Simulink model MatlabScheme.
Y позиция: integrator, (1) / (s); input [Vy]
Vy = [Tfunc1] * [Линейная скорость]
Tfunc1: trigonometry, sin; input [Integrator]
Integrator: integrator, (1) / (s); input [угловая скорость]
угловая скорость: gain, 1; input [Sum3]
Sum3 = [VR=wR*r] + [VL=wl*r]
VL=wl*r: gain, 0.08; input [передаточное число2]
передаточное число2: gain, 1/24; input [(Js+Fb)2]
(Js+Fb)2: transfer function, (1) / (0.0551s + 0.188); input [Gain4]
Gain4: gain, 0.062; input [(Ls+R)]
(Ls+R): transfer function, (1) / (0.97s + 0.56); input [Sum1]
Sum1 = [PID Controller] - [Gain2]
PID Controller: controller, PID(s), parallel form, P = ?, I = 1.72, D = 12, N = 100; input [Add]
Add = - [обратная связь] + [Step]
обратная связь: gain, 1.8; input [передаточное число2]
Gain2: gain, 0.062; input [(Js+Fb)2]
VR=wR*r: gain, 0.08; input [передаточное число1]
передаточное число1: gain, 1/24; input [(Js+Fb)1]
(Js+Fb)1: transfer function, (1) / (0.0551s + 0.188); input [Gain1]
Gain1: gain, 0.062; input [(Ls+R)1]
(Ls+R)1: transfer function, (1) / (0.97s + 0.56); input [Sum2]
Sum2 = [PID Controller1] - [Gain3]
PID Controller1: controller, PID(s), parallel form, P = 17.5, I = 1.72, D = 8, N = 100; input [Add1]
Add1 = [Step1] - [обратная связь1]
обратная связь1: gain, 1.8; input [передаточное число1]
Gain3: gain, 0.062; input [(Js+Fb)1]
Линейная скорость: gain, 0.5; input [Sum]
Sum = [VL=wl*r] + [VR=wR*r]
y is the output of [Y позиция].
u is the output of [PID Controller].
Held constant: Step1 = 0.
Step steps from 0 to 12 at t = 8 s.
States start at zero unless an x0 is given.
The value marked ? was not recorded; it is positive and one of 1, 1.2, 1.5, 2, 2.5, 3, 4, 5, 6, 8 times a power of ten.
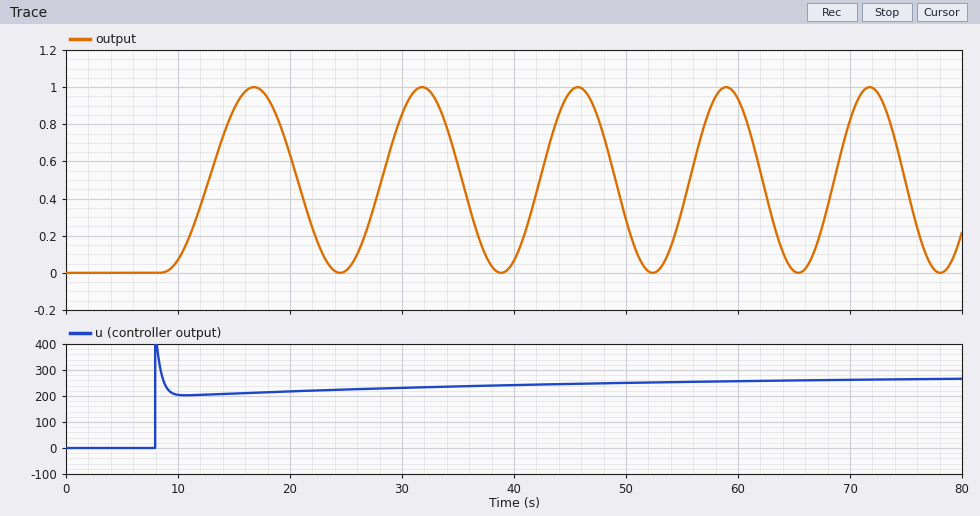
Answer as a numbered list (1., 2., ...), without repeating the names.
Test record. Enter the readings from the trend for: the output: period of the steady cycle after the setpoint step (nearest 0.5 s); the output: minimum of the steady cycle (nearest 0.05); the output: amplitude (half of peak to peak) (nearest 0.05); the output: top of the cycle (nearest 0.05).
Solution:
1. 13.0 s
2. 0.00
3. 0.50
4. 1.00
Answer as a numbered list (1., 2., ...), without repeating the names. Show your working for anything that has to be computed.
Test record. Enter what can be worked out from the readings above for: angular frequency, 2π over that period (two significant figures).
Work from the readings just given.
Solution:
1. 2π / 13 = 0.48 rad/s
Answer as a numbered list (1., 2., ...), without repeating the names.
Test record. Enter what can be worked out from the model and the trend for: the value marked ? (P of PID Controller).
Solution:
1. 50
